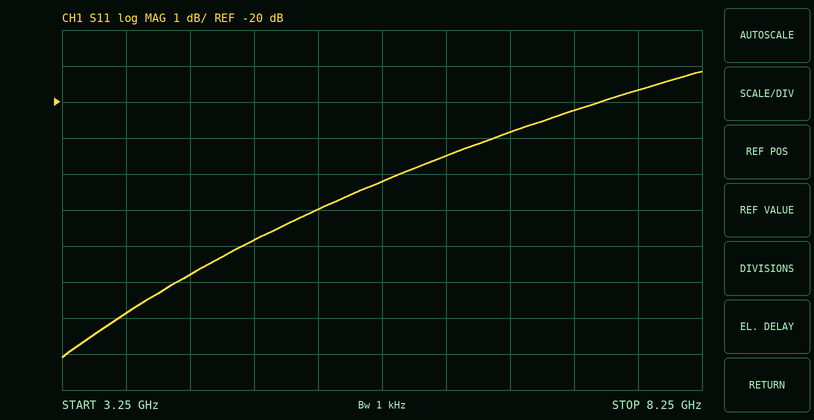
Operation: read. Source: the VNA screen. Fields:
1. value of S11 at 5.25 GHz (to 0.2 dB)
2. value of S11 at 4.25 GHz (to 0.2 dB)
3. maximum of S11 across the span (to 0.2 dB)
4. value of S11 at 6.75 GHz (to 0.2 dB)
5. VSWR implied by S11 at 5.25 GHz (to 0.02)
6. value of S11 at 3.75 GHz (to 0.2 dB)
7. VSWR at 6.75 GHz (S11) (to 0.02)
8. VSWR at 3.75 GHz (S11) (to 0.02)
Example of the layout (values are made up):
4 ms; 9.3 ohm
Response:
-23.0 dB; -24.8 dB; -19.2 dB; -20.8 dB; 1.16; -25.8 dB; 1.20; 1.10
